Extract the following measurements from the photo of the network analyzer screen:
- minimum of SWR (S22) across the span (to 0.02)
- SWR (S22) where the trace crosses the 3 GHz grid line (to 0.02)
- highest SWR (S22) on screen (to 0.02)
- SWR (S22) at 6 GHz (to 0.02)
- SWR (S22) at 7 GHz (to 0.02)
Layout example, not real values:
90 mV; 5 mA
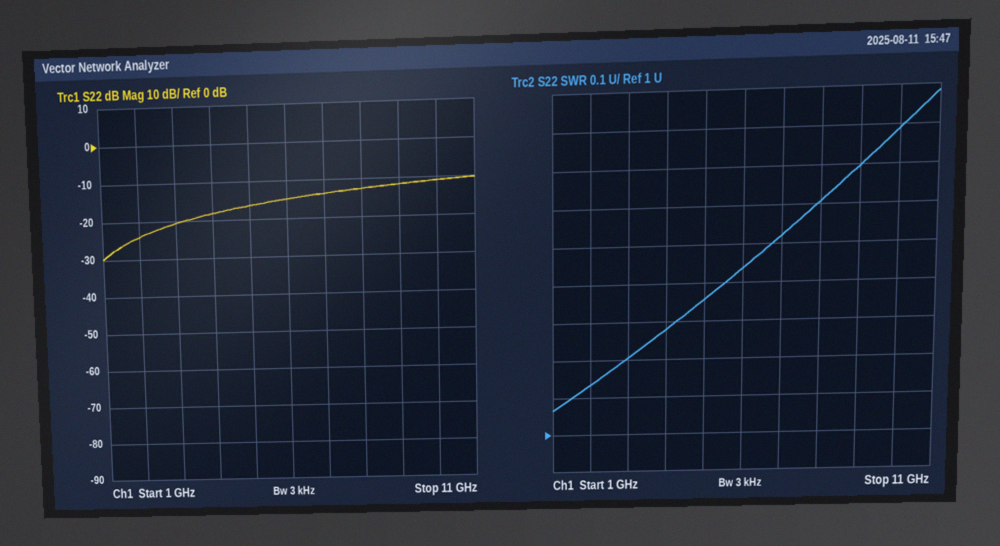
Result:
1.06; 1.20; 1.88; 1.44; 1.52
